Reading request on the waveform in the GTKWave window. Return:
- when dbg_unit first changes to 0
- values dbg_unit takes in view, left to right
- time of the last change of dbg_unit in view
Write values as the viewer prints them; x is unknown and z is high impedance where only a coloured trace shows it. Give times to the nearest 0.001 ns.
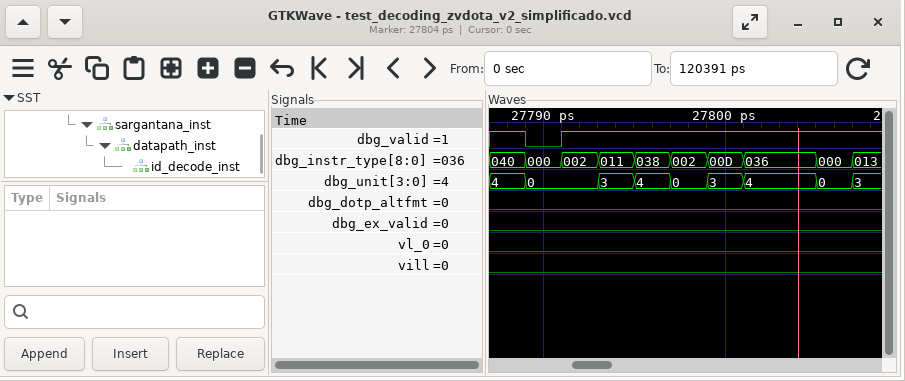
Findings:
27.789 ns
4, 0, 3, 4, 0, 3, 4, 0, 3
27.807 ns
